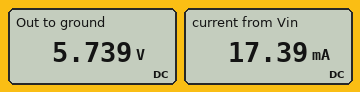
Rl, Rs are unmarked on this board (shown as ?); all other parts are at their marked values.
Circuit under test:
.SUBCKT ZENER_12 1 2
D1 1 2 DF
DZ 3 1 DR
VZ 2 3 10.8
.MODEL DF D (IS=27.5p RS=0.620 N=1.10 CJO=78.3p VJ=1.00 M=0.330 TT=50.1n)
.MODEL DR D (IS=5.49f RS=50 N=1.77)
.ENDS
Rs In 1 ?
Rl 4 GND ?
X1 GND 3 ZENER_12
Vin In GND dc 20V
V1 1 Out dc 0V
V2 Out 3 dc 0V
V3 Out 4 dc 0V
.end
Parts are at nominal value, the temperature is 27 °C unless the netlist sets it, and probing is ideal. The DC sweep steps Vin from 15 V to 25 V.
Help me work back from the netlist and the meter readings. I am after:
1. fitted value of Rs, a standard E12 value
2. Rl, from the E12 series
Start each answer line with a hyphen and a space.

- 820 Ω
- 330 Ω
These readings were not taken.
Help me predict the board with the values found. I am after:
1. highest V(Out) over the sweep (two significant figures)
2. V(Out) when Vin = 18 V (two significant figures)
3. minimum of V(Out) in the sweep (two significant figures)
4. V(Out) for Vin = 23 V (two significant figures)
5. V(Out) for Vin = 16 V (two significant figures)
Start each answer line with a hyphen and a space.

- 7.2 V
- 5.2 V
- 4.3 V
- 6.6 V
- 4.6 V
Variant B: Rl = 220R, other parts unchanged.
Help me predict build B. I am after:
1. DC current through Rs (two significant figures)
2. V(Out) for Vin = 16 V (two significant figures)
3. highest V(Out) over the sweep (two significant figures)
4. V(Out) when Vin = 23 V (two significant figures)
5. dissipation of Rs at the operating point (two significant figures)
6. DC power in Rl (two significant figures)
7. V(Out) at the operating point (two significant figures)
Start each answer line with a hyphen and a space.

- 19 mA
- 3.4 V
- 5.3 V
- 4.9 V
- 300 mW
- 81 mW
- 4.2 V
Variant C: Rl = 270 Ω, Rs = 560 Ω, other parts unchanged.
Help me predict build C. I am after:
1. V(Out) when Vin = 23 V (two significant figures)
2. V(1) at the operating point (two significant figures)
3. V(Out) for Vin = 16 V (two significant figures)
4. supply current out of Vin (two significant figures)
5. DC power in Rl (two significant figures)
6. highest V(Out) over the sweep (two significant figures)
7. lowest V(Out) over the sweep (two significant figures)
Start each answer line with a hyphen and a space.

- 7.5 V
- 6.5 V
- 5.2 V
- 24 mA
- 160 mW
- 8.1 V
- 4.9 V
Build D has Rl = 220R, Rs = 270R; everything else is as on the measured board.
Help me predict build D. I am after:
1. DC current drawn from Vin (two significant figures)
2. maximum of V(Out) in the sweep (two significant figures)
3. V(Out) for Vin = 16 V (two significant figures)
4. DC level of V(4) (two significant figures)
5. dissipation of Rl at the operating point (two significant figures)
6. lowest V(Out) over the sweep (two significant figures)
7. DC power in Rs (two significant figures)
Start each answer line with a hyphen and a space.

- 41 mA
- 11 V
- 7.2 V
- 9.0 V
- 370 mW
- 6.7 V
- 450 mW
